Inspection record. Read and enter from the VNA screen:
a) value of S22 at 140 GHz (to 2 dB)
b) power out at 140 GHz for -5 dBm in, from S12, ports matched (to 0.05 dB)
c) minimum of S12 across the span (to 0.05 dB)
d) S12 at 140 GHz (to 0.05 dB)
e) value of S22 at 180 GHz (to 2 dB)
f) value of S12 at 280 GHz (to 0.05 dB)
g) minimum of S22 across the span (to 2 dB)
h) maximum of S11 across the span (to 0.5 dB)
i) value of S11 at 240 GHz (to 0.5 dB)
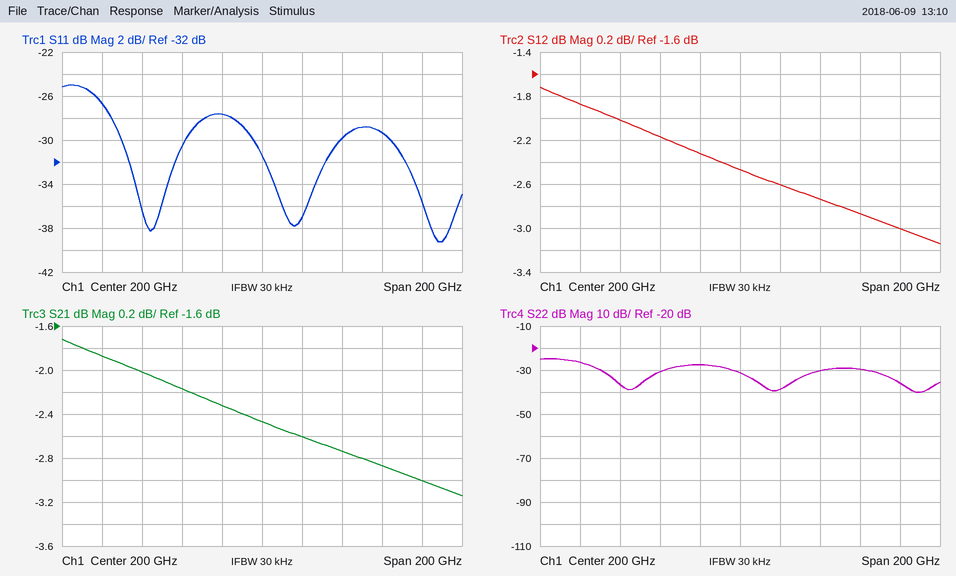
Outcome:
-36 dB
-7.00 dBm
-3.15 dB
-2.00 dB
-28 dB
-3.00 dB
-40 dB
-25.0 dB
-30.0 dB
